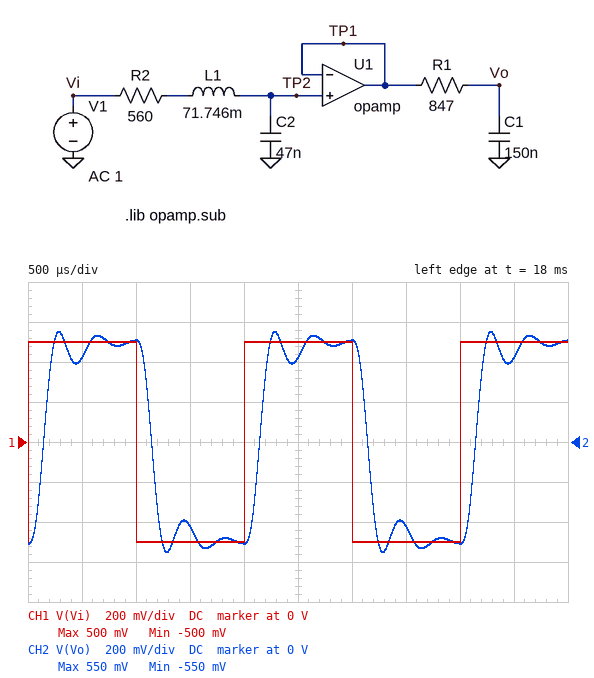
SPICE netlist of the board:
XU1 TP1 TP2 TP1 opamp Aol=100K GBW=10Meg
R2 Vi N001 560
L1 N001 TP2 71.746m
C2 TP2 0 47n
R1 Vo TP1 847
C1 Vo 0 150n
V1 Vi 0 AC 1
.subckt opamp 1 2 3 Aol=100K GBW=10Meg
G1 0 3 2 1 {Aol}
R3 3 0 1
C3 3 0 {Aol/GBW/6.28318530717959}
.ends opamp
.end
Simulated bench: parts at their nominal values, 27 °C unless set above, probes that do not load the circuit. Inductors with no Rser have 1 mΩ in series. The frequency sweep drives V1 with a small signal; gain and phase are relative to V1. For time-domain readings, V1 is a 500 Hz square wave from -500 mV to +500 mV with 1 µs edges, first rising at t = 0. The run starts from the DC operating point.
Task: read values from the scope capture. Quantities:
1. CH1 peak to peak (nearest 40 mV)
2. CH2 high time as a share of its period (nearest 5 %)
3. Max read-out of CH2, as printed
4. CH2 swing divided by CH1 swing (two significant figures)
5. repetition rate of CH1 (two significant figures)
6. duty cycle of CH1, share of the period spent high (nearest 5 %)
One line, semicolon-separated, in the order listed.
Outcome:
1.00 V; 50 %; 550 mV; 1.1; 500 Hz; 50 %
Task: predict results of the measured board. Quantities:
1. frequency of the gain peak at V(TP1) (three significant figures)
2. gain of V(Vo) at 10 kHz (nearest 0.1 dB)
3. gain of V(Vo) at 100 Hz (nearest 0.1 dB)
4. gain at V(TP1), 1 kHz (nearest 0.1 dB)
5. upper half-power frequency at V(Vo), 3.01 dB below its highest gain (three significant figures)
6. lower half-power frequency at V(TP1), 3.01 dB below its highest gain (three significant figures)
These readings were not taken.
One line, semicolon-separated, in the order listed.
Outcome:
2.60 kHz; -40.0 dB; 0 dB; 1.1 dB; 3.01 kHz; 1.85 kHz
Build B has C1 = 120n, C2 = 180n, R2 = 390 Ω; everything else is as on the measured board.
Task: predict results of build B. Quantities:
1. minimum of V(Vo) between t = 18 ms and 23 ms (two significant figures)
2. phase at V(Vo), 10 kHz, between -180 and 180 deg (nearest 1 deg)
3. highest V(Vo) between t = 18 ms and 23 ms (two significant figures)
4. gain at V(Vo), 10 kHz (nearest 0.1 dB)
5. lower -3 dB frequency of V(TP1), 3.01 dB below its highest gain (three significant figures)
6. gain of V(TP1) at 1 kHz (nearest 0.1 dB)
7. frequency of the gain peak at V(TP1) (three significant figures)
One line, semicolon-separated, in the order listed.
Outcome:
-740 mV; 104 deg; 740 mV; -50.2 dB; 659 Hz; 3.6 dB; 1.26 kHz
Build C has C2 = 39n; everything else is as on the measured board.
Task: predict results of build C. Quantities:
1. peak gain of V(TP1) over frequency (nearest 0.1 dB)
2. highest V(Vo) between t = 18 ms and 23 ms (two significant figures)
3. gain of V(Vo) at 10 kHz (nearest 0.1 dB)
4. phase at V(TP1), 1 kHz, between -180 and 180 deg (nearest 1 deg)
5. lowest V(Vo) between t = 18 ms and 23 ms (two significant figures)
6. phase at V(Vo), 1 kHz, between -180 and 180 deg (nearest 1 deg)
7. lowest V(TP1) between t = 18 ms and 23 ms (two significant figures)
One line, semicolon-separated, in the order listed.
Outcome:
7.9 dB; 530 mV; -38.2 dB; -9 deg; -530 mV; -47 deg; -1.0 V
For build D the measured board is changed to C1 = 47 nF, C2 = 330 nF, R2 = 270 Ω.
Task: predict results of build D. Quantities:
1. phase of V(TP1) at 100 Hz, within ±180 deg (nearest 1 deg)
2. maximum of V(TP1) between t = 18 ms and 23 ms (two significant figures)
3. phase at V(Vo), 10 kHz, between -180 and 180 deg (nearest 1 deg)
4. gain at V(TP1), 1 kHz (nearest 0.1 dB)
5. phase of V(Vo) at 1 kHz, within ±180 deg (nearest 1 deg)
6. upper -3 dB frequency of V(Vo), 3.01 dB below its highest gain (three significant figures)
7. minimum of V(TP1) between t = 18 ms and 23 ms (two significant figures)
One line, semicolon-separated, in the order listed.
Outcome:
-3 deg; 840 mV; 115 deg; 5.0 dB; -97 deg; 1.21 kHz; -840 mV
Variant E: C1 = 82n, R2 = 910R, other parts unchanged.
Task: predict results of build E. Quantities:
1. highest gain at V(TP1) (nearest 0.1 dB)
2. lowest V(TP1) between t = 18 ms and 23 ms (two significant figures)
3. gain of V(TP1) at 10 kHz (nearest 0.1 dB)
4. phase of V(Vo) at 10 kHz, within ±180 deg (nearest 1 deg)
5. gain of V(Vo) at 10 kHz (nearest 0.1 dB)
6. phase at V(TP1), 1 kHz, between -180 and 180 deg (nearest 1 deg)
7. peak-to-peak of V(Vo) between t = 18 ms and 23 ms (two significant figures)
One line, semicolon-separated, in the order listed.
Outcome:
3.3 dB; -790 mV; -22.0 dB; 115 deg; -35.0 dB; -17 deg; 1.3 V
